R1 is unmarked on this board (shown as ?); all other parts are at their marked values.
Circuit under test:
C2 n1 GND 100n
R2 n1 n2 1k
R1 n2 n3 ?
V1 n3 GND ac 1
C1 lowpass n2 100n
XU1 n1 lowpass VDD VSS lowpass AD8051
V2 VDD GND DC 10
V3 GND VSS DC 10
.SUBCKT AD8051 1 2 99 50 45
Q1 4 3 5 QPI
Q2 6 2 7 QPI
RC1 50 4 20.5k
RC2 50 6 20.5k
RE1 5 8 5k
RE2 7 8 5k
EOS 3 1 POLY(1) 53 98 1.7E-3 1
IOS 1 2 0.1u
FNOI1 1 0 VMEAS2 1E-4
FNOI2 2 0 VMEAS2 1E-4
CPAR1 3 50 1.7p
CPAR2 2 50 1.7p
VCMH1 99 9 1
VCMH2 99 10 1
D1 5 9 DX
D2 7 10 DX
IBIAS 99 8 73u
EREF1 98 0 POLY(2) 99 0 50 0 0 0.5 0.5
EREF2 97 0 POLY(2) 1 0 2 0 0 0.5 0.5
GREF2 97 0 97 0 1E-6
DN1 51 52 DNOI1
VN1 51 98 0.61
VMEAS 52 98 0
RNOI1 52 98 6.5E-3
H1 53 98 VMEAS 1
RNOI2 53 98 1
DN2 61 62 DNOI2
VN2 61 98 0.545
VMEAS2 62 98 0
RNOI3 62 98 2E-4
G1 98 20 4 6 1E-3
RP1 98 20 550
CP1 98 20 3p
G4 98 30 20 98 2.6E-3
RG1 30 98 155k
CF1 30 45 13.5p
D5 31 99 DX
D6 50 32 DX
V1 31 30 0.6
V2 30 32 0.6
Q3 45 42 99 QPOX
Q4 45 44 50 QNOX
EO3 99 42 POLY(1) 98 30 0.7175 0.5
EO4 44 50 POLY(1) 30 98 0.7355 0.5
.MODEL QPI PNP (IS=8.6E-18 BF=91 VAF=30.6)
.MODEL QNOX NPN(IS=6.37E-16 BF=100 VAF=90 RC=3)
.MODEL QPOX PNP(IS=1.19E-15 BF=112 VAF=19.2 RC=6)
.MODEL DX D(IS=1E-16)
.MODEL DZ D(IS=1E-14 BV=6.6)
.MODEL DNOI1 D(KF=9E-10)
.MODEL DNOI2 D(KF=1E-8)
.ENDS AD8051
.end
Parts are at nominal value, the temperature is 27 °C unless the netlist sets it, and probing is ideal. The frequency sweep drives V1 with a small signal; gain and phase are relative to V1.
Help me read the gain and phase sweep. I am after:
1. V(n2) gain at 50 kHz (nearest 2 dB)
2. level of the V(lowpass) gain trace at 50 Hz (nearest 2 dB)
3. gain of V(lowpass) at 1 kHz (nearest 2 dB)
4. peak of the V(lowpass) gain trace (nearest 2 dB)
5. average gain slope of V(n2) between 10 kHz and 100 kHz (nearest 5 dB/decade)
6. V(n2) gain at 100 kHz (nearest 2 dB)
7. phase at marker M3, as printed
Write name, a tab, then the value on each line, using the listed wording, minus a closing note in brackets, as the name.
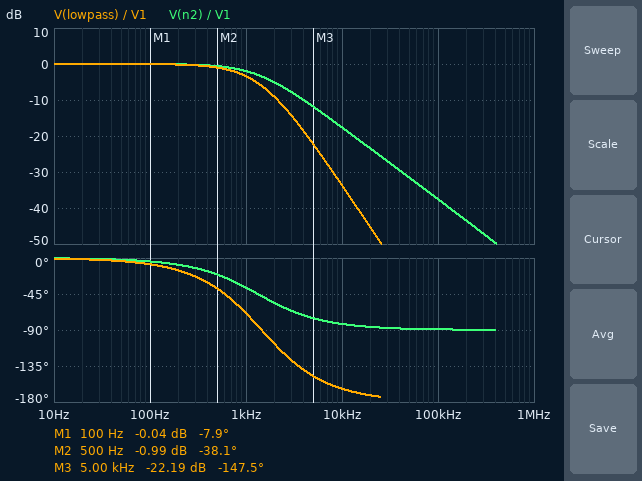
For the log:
V(n2) gain at 50 kHz	-32 dB
level of the V(lowpass) gain trace at 50 Hz	0 dB
gain of V(lowpass) at 1 kHz	-4 dB
peak of the V(lowpass) gain trace	0 dB
average gain slope of V(n2) between 10 kHz and 100 kHz	-20 dB/decade
V(n2) gain at 100 kHz	-38 dB
phase at marker M3, as printed	-147.5 deg
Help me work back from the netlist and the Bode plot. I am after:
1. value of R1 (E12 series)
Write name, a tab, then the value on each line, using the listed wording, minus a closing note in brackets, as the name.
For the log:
value of R1	1.2 kΩ
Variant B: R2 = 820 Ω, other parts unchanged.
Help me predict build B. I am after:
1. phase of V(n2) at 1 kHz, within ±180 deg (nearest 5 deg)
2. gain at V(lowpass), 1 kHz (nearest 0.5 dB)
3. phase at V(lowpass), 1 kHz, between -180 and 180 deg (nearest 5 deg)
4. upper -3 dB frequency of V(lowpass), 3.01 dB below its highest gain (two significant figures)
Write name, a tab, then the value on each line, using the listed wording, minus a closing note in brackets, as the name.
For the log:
phase of V(n2) at 1 kHz, within ±180 deg	-35 deg
gain at V(lowpass), 1 kHz	-3.0 dB
phase at V(lowpass), 1 kHz, between -180 and 180 deg	-65 deg
upper -3 dB frequency of V(lowpass), 3.01 dB below its highest gain	1.0 kHz
